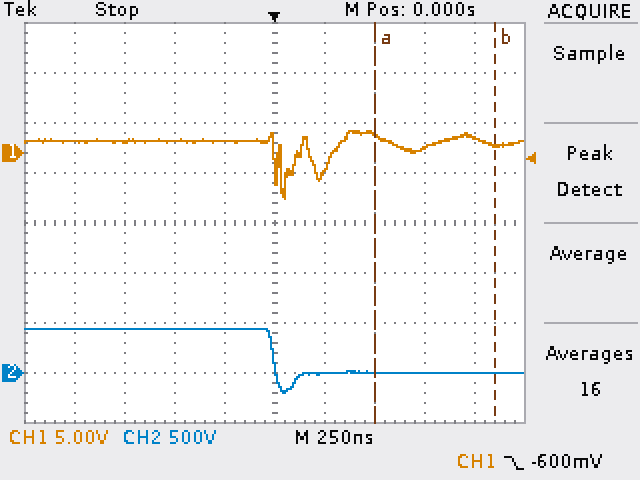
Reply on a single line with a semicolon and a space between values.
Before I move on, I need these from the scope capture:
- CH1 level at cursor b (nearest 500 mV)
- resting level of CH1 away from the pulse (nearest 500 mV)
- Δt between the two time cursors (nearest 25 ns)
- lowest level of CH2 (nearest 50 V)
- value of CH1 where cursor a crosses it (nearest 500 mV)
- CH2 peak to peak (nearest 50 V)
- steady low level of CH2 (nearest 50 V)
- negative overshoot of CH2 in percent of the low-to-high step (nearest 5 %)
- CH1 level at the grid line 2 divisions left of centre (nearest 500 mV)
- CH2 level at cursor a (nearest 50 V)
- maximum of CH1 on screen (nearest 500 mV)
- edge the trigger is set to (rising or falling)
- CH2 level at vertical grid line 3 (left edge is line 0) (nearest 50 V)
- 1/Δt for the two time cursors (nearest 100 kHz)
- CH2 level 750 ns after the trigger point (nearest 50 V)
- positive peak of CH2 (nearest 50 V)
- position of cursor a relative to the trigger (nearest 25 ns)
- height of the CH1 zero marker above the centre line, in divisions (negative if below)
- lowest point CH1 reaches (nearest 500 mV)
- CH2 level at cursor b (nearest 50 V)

1.0 V; 1.0 V; 600 ns; -200 V; 1.5 V; 650 V; 0 V; 45 %; 1.0 V; 0 V; 2.0 V; falling; 450 V; 1.7 MHz; 0 V; 450 V; +500 ns; +1.4 div; -4.5 V; 0 V
